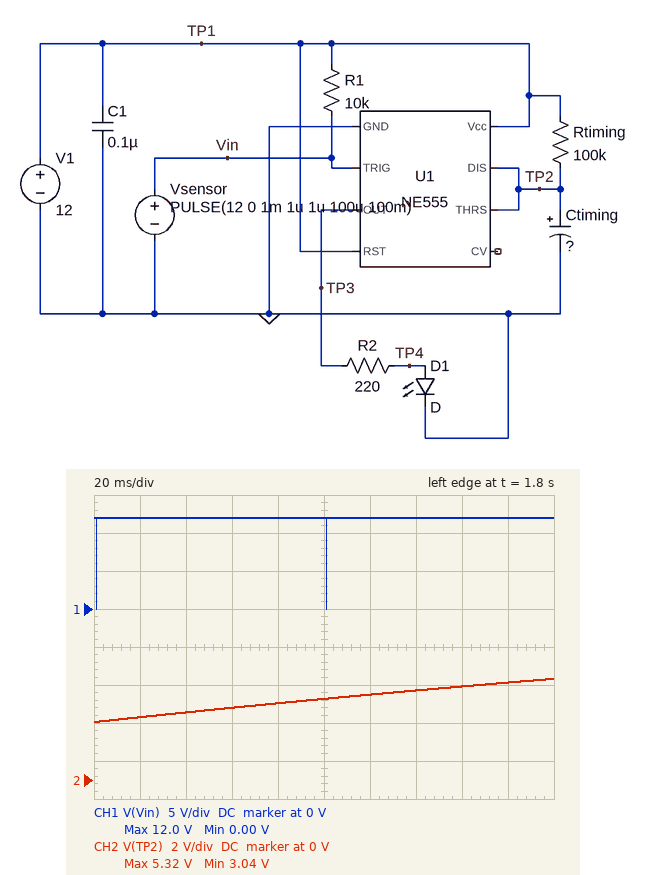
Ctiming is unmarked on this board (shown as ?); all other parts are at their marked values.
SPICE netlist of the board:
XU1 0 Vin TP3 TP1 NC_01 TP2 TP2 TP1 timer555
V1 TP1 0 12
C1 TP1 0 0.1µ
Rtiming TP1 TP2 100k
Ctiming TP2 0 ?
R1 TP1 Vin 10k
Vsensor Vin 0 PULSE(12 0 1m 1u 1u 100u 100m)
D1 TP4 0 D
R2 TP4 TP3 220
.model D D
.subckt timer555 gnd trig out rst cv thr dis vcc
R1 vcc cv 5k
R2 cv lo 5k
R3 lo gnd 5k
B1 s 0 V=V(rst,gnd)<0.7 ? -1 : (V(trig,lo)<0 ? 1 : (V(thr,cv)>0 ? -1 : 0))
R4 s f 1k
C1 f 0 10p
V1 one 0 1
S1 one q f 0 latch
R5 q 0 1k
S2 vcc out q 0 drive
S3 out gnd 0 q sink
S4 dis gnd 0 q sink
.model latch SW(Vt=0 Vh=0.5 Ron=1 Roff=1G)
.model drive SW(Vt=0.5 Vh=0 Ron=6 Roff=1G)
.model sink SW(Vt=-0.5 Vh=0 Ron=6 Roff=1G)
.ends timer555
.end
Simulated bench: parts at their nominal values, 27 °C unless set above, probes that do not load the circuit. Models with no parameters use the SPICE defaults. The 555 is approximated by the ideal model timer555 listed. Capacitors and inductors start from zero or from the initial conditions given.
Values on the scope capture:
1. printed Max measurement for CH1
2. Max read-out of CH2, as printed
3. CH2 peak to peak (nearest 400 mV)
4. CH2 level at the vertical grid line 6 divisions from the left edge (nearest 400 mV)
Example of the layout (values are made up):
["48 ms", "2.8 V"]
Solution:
["12.0 V", "5.32 V", "2.4 V", "4.4 V"]
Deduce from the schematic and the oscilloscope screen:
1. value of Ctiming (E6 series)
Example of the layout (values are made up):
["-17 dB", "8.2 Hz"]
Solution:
["6.8 µF"]
